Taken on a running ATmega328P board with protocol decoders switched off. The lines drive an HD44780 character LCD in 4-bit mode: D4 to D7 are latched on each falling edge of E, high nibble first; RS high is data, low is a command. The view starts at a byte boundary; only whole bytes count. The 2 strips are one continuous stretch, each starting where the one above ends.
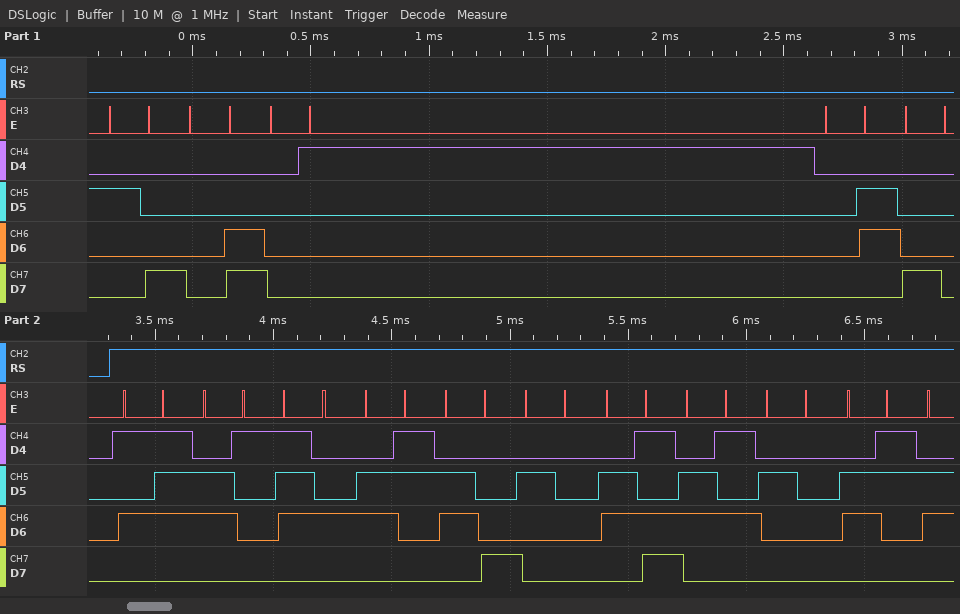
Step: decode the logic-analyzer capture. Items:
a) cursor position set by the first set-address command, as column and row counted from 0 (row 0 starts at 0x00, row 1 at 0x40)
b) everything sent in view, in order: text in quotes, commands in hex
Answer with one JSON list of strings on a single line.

["column 0, row 0", "0x28 0x0C 0x01 0x06 0x80 \"Watch me c\""]
